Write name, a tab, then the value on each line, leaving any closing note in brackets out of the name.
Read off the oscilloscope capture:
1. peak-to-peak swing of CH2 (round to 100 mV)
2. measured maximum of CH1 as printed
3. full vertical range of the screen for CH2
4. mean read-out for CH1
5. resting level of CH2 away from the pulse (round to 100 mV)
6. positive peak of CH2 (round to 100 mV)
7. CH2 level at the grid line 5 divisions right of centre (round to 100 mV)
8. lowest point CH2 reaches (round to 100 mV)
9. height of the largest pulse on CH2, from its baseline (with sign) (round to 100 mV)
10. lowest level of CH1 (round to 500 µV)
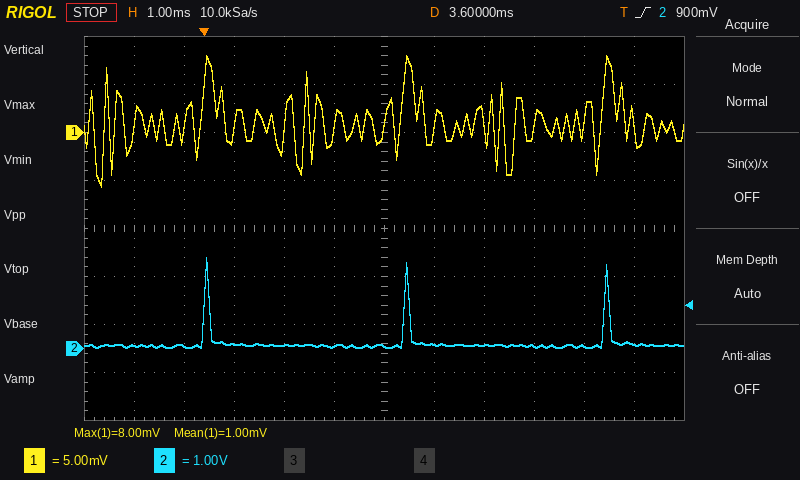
peak-to-peak swing of CH2	1.9 V
measured maximum of CH1 as printed	8.00 mV
full vertical range of the screen for CH2	8 V
mean read-out for CH1	1.00 mV
resting level of CH2 away from the pulse	100 mV
positive peak of CH2	1.9 V
CH2 level at the grid line 5 divisions right of centre	100 mV
lowest point CH2 reaches	0.0 V
height of the largest pulse on CH2, from its baseline (with sign)	+1.8 V
lowest level of CH1	-5.5 mV
